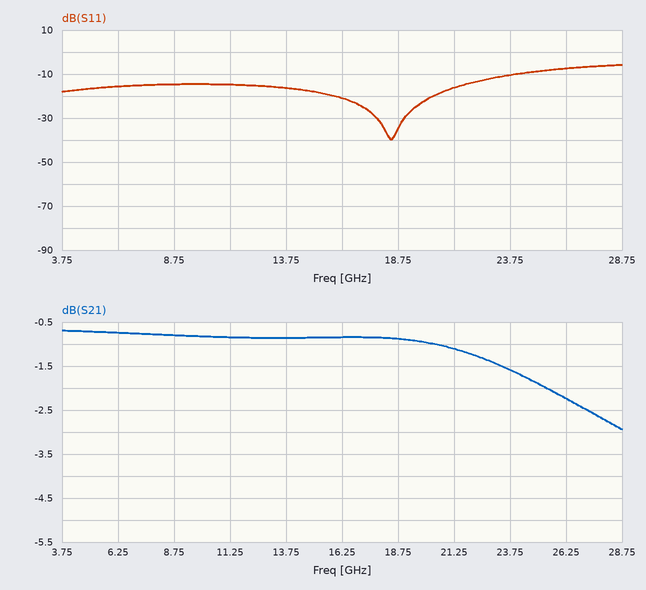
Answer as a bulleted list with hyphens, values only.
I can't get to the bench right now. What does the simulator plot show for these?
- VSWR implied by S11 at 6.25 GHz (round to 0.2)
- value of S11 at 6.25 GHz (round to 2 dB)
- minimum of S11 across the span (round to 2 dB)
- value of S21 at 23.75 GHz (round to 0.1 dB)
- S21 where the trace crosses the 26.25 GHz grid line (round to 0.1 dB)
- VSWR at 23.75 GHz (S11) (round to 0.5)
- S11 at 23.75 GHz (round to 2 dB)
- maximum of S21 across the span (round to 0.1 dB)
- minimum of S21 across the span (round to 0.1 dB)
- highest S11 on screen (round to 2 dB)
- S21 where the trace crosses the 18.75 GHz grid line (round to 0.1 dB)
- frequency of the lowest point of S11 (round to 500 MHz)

- 1.4
- -16 dB
- -40 dB
- -1.6 dB
- -2.2 dB
- 2.0
- -10 dB
- -0.7 dB
- -2.9 dB
- -6 dB
- -0.9 dB
- 18.5 GHz
